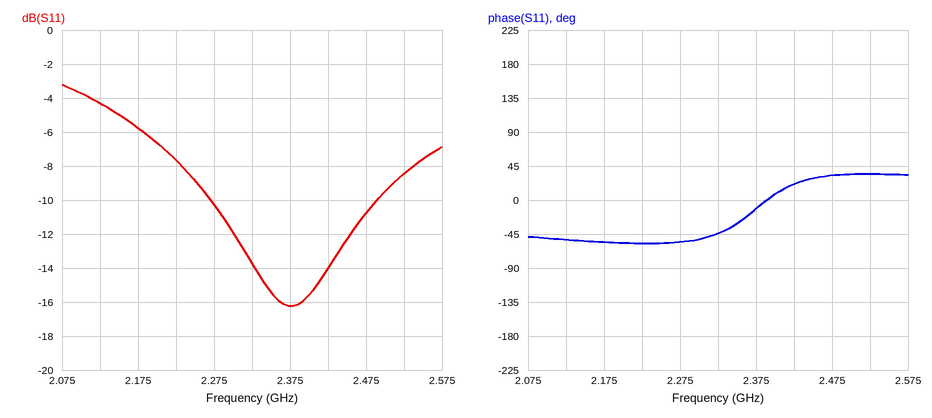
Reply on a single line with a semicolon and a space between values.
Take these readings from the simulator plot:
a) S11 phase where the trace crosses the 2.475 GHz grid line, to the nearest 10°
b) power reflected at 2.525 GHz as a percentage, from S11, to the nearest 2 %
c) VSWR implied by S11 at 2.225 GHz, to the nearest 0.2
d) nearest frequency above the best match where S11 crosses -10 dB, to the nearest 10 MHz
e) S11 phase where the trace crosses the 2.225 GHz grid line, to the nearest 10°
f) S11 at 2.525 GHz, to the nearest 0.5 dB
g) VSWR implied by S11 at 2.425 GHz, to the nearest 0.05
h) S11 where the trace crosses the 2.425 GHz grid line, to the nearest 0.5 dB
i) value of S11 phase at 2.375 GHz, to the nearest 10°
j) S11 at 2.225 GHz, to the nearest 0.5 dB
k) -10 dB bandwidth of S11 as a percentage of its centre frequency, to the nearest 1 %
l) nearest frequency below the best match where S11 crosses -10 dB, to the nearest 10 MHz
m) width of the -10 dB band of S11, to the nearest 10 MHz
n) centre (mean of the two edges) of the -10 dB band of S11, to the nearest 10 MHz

30°; 14 %; 2.4; 2.49 GHz; -60°; -8.5 dB; 1.50; -14.0 dB; -10°; -7.5 dB; 9 %; 2.27 GHz; 220 MHz; 2.38 GHz
